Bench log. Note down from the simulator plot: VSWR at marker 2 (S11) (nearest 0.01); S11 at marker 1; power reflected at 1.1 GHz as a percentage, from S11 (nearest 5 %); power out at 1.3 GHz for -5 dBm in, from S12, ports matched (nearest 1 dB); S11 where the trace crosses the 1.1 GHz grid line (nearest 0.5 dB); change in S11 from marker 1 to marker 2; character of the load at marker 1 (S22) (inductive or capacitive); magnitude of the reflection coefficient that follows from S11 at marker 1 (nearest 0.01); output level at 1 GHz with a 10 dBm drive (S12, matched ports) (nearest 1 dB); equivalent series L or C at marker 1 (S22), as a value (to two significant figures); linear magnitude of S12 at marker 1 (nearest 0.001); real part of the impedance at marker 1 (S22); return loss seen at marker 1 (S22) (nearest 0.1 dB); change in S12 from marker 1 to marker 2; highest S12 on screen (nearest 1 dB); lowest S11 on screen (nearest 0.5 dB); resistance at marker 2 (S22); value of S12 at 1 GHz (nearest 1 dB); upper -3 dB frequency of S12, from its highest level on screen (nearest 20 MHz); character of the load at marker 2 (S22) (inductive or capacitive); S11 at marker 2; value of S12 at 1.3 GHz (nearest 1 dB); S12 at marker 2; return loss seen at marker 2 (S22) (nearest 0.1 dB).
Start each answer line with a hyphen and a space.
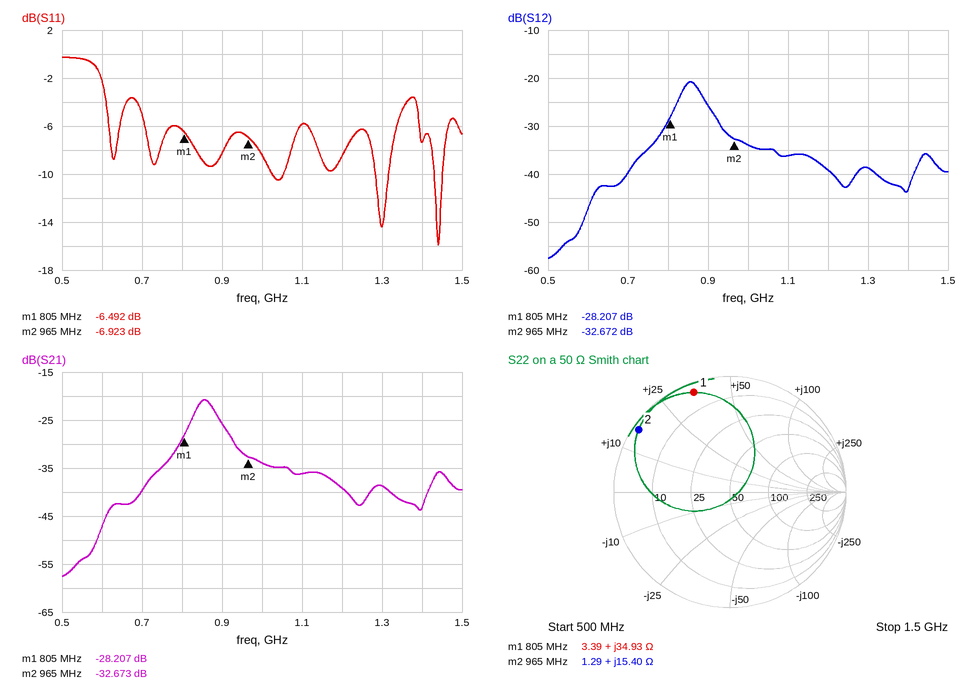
- 2.64
- -6.492 dB
- 25 %
- -44 dBm
- -6.0 dB
- -0.431 dB
- inductive
- 0.47
- -24 dBm
- 6.9 nH
- 0.039
- 3.39 Ω
- 0.8 dB
- -4.465 dB
- -21 dB
- -16.0 dB
- 1.29 Ω
- -34 dB
- 880 MHz
- inductive
- -6.923 dB
- -39 dB
- -32.672 dB
- 0.4 dB
